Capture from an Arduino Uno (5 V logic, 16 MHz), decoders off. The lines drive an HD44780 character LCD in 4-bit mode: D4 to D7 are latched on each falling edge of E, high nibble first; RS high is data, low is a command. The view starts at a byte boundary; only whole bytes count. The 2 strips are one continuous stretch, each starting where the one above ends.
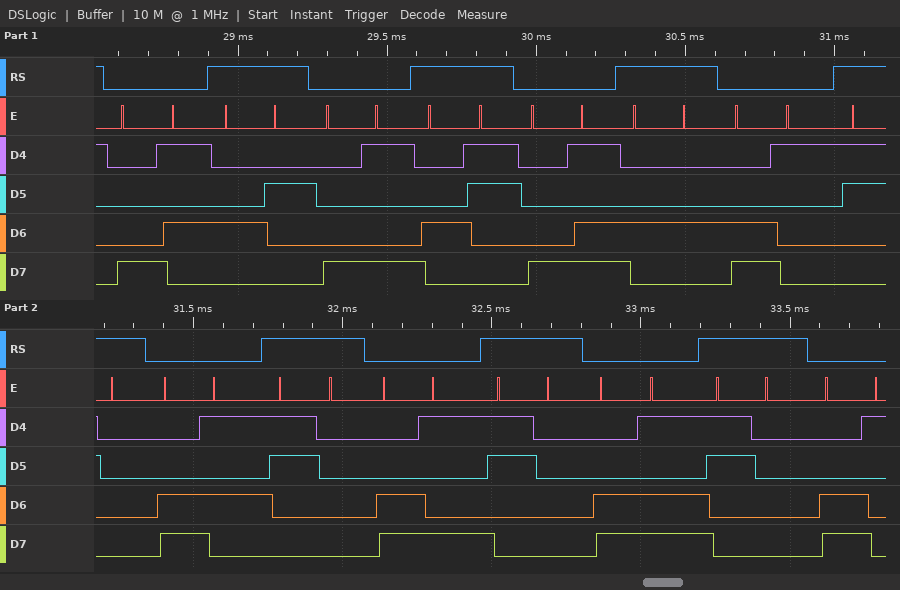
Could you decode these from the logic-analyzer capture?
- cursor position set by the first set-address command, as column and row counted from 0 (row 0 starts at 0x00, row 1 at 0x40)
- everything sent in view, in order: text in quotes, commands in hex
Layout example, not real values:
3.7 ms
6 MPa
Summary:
column 5, row 0
0x85 "B" 0x89 "C" 0x8D "D" 0xC1 "0" 0xC5 "0" 0xC9 "0" 0xCD "0" 0xC1
